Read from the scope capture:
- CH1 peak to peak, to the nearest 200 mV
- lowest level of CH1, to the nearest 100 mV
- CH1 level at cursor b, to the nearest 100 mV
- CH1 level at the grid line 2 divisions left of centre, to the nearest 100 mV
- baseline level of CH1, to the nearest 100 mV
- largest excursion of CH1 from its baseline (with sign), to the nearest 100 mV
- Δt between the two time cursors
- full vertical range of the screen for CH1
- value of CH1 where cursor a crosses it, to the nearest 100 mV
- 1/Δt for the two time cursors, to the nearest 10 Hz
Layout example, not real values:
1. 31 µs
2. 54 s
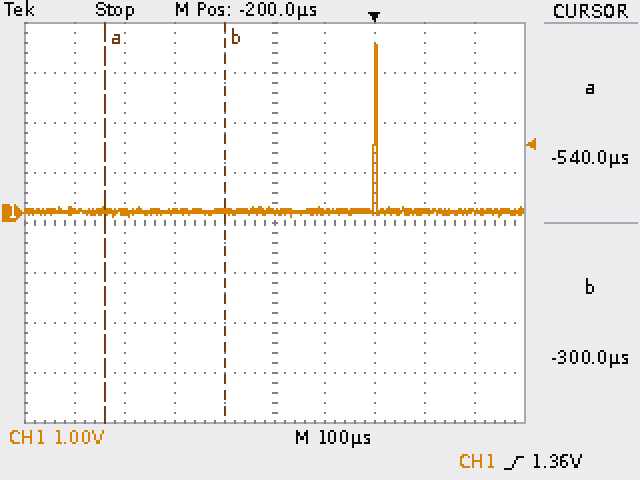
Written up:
1. 3.4 V
2. -100 mV
3. 0.0 V
4. 0.0 V
5. 0.0 V
6. +3.3 V
7. 240 µs
8. 8 V
9. 0.0 V
10. 4.17 kHz
